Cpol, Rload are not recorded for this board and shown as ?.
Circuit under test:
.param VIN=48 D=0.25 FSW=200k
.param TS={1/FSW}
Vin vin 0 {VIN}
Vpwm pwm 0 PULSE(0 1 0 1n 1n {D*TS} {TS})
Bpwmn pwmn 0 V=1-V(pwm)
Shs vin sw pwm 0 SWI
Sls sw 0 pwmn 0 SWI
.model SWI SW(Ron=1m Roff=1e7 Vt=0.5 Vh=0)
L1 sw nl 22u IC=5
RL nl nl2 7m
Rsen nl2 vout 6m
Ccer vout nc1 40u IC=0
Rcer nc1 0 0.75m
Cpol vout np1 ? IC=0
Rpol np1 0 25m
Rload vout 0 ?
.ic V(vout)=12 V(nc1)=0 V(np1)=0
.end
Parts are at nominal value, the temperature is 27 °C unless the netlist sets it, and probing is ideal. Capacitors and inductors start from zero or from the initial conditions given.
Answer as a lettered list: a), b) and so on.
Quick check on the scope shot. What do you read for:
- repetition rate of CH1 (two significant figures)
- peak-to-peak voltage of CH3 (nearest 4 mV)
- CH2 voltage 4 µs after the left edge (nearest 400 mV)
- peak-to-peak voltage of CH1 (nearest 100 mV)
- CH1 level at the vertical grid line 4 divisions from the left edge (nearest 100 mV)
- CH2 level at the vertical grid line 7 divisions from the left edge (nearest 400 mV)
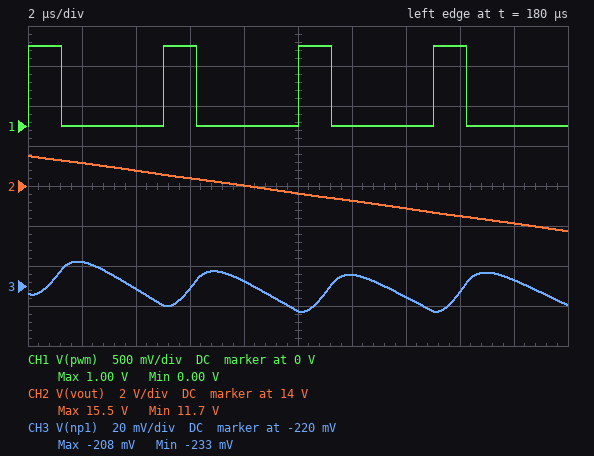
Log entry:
a) 200 kHz
b) 24 mV
c) 14.8 V
d) 1.0 V
e) 0 V
f) 12.8 V
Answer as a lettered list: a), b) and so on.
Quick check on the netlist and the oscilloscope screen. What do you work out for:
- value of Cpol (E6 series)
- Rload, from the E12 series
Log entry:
a) 47 µF
b) 3.9 Ω
